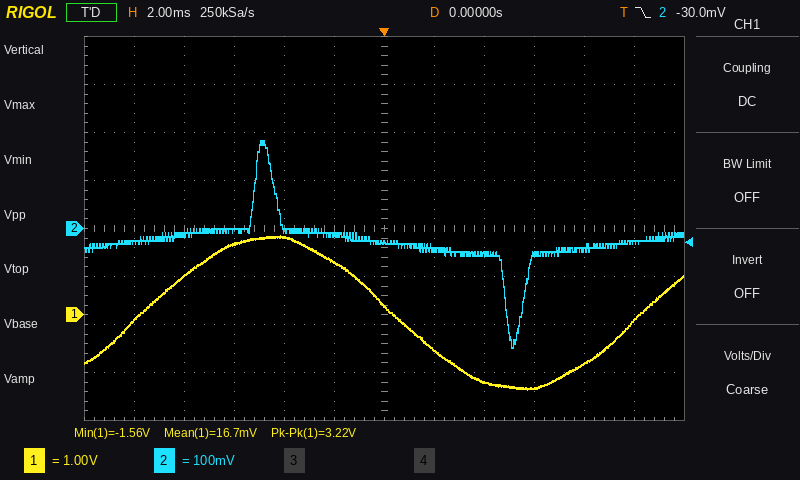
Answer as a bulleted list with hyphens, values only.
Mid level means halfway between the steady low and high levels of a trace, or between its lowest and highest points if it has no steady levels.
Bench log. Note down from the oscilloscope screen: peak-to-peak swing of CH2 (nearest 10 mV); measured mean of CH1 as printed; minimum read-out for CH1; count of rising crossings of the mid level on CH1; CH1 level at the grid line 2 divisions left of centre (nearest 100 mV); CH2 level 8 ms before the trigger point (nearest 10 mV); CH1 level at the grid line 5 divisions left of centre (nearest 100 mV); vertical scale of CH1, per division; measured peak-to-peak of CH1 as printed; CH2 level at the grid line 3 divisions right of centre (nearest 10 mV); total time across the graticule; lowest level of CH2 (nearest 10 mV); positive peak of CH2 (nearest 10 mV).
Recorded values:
- 430 mV
- 16.7 mV
- -1.56 V
- 2
- 1.6 V
- -10 mV
- -100 mV
- 1 V
- 3.22 V
- -60 mV
- 24 ms
- -250 mV
- 180 mV
